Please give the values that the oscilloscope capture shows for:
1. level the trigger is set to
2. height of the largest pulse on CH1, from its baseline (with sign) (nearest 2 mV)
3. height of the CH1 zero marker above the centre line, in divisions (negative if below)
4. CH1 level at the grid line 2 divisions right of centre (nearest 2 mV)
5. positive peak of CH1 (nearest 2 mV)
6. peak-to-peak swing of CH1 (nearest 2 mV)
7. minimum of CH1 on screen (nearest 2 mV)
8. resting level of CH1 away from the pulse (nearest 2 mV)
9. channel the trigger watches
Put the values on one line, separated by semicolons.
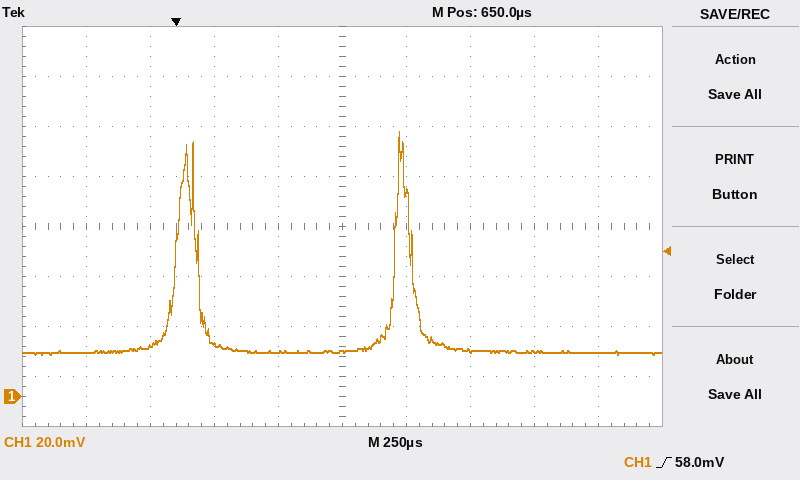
58.0 mV; +88 mV; -3.4 div; 18 mV; 106 mV; 90 mV; 16 mV; 18 mV; CH1
